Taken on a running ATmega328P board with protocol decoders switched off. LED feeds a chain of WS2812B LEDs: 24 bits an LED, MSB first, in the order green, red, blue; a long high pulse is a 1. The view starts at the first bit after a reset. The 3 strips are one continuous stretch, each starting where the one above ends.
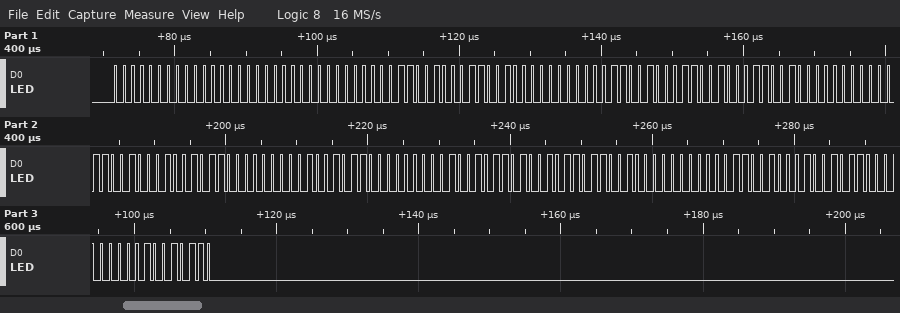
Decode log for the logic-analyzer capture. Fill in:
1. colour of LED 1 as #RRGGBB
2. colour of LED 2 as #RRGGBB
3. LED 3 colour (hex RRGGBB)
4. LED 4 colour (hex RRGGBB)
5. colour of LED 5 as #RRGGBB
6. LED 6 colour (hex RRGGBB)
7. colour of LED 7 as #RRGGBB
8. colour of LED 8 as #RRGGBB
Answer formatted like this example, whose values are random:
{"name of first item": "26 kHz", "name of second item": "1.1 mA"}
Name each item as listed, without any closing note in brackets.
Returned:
{"colour of LED 1 as #RRGGBB": "#000000", "colour of LED 2 as #RRGGBB": "#C800C8", "LED 3 colour": "#C800C8", "LED 4 colour": "#00C8C8", "colour of LED 5 as #RRGGBB": "#009696", "LED 6 colour": "#960096", "colour of LED 7 as #RRGGBB": "#00C8C8", "colour of LED 8 as #RRGGBB": "#009696"}
